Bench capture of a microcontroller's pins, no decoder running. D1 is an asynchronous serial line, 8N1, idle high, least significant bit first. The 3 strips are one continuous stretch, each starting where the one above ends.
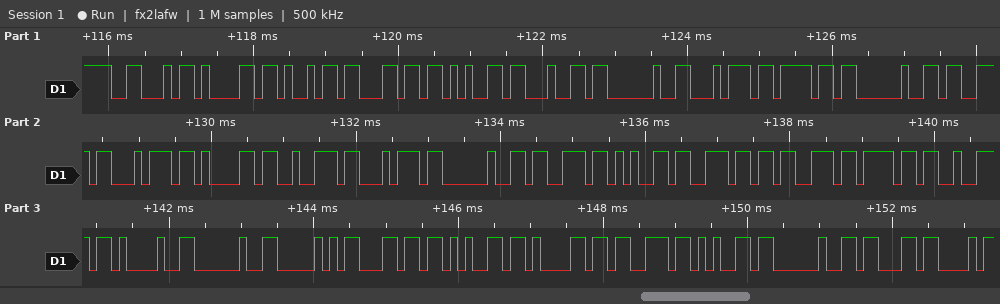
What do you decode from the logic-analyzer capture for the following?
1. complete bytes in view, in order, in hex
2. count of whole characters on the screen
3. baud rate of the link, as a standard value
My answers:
46 61 69 6C 65 64 20 74 6F 20 73 74 61 72 74 20 73 65 6E 73 6F 72 21 20 50 6C 65 61 73 65 20 63
32
9600 baud
